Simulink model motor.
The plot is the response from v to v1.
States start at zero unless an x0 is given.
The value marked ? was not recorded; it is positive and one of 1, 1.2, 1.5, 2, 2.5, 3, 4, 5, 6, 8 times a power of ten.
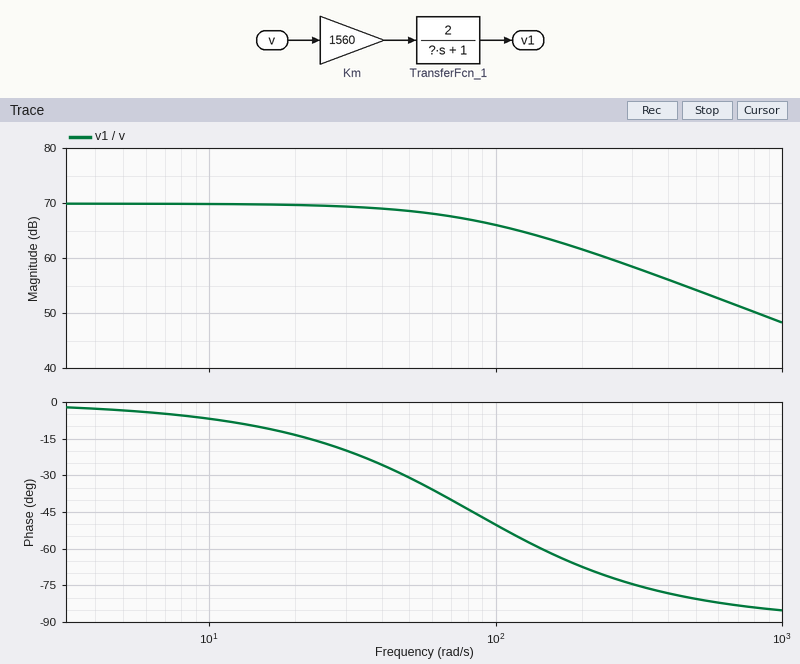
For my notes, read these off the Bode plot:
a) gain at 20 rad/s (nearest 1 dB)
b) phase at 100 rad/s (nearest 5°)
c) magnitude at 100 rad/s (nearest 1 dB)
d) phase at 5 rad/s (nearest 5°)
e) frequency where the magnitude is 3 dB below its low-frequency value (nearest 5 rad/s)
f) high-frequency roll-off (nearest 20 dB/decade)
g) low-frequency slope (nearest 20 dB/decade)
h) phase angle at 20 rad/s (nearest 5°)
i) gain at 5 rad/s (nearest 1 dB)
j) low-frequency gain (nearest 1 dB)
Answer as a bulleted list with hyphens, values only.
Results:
- 70 dB
- -50°
- 66 dB
- -5°
- 85 rad/s
- -20 dB/decade
- 0 dB/decade
- -15°
- 70 dB
- 70 dB
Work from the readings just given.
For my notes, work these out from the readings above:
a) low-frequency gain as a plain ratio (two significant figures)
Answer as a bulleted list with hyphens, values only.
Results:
- 3200
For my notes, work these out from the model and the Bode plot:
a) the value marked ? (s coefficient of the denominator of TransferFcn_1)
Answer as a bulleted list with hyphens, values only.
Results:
- 0.012
